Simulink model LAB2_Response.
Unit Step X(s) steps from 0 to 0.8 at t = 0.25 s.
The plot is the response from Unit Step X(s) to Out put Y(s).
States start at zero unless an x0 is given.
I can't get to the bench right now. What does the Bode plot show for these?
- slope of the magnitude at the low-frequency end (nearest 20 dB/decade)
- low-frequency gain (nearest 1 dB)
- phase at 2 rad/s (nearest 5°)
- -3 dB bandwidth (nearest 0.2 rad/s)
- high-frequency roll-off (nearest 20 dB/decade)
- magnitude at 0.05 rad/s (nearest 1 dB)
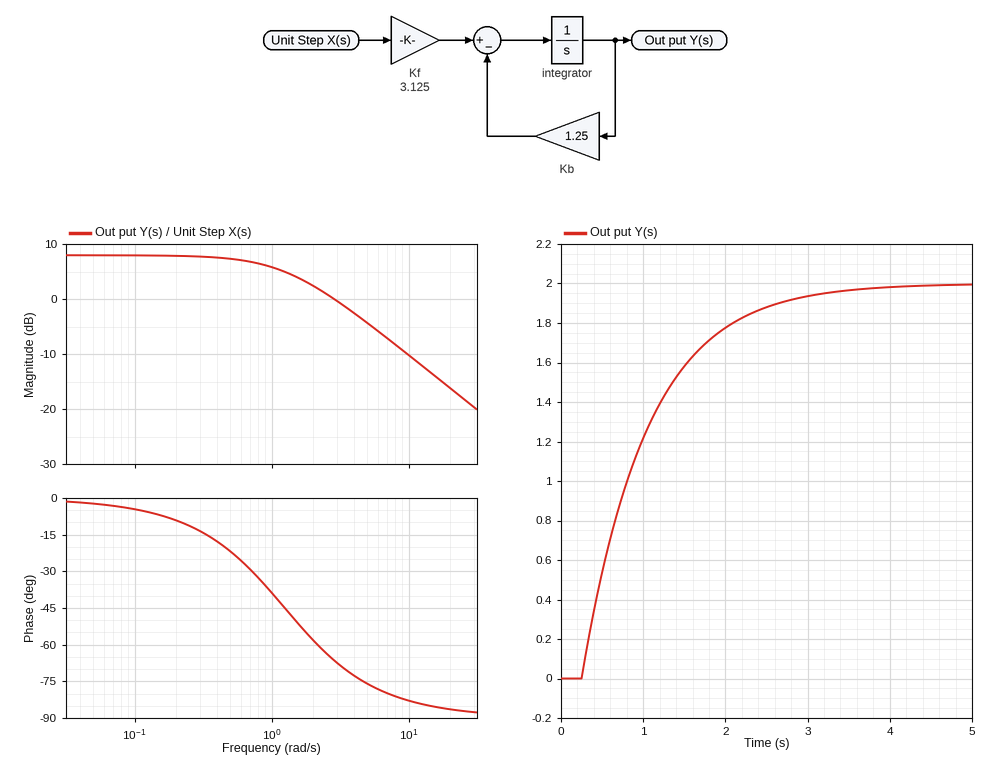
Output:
0 dB/decade
8 dB
-60°
1.2 rad/s
-20 dB/decade
8 dB
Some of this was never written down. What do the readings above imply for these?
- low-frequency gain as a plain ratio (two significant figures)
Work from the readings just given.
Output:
2.5
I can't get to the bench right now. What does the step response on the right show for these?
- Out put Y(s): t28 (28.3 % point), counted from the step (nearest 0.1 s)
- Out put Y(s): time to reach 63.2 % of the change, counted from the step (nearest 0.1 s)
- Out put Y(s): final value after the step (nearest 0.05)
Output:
0.3 s
0.8 s
2.00
